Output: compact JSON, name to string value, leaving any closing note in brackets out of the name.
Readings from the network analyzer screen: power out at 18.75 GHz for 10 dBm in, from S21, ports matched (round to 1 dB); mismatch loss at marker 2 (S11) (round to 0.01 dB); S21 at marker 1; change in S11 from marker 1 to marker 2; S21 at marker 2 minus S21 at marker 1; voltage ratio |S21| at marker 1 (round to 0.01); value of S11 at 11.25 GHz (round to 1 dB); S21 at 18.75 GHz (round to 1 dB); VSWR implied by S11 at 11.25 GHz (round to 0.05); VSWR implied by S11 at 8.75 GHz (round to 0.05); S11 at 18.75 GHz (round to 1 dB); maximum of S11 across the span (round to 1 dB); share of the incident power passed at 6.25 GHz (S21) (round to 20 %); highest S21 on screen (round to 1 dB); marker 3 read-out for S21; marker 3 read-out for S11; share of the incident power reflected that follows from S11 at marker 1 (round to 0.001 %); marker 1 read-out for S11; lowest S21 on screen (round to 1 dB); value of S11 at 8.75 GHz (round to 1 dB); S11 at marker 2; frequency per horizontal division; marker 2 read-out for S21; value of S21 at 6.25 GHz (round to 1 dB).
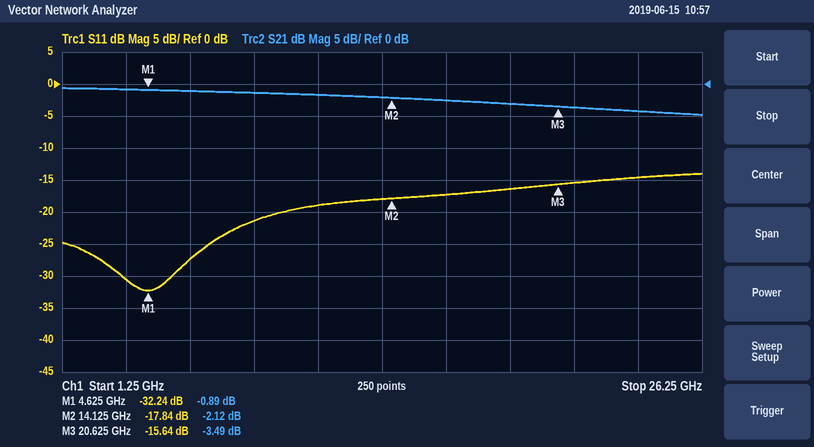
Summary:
{"power out at 18.75 GHz for 10 dBm in, from S21, ports matched": "7 dBm", "mismatch loss at marker 2 (S11)": "0.07 dB", "S21 at marker 1": "-0.89 dB", "change in S11 from marker 1 to marker 2": "14.40 dB", "S21 at marker 2 minus S21 at marker 1": "-1.23 dB", "voltage ratio |S21| at marker 1": "0.90", "value of S11 at 11.25 GHz": "-19 dB", "S21 at 18.75 GHz": "-3 dB", "VSWR implied by S11 at 11.25 GHz": "1.25", "VSWR implied by S11 at 8.75 GHz": "1.20", "S11 at 18.75 GHz": "-16 dB", "maximum of S11 across the span": "-14 dB", "share of the incident power passed at 6.25 GHz (S21)": "80 %", "highest S21 on screen": "-1 dB", "marker 3 read-out for S21": "-3.49 dB", "marker 3 read-out for S11": "-15.64 dB", "share of the incident power reflected that follows from S11 at marker 1": "0.060 %", "marker 1 read-out for S11": "-32.24 dB", "lowest S21 on screen": "-5 dB", "value of S11 at 8.75 GHz": "-21 dB", "S11 at marker 2": "-17.84 dB", "frequency per horizontal division": "2.5 GHz", "marker 2 read-out for S21": "-2.12 dB", "value of S21 at 6.25 GHz": "-1 dB"}
